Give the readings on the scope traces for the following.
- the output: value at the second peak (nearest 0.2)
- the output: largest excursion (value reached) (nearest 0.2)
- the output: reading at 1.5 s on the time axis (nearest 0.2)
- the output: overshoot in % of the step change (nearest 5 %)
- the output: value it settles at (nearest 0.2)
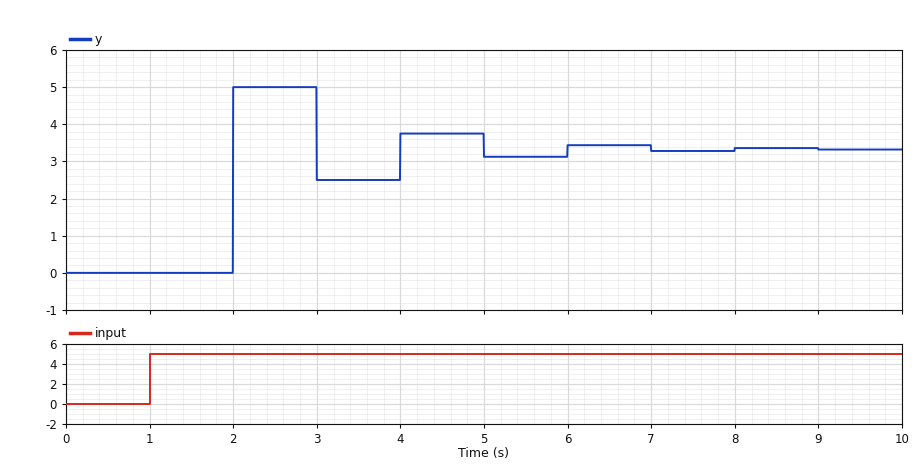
3.8
5.0
0.0
50 %
3.4
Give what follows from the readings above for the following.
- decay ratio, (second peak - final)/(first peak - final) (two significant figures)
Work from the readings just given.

0.25
